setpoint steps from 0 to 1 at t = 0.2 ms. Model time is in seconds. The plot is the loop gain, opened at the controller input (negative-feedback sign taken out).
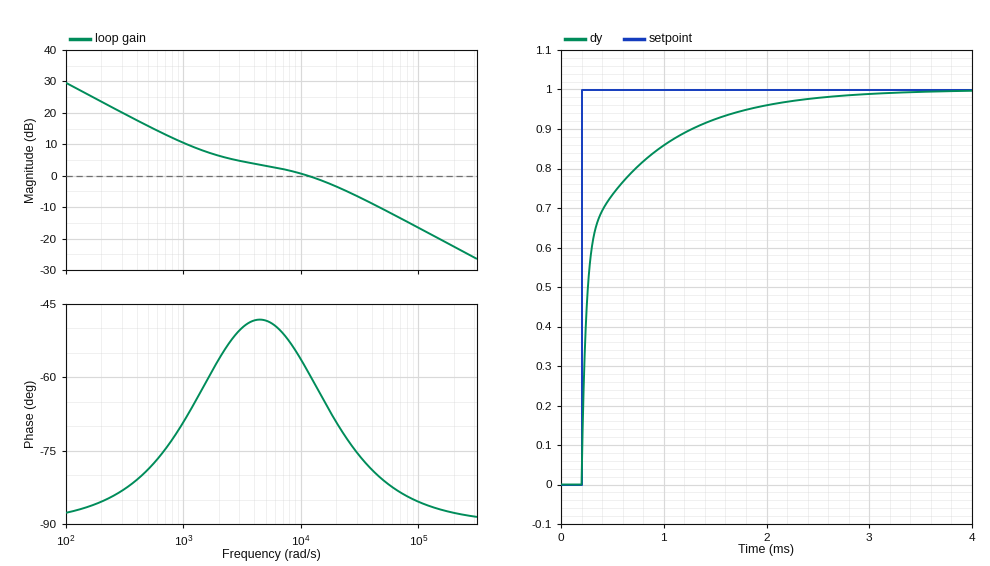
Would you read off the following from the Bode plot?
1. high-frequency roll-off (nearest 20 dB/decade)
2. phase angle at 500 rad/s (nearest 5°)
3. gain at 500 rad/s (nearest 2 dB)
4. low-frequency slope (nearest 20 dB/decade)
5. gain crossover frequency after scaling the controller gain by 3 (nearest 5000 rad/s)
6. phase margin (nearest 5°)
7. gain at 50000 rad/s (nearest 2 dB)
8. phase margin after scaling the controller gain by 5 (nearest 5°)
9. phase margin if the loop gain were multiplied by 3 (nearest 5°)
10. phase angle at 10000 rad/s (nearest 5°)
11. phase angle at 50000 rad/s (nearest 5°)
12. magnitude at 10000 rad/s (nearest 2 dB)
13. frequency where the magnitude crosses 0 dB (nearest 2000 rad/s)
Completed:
-20 dB/decade
-80°
16 dB
-20 dB/decade
45000 rad/s
120°
-10 dB
95°
100°
-55°
-80°
0 dB
12000 rad/s
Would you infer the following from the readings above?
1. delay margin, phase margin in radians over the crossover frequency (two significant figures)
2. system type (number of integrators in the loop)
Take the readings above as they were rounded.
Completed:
0.00017 s
1
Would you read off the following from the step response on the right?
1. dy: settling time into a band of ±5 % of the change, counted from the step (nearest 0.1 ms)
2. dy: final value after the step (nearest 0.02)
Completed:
1.6 ms
1.00
